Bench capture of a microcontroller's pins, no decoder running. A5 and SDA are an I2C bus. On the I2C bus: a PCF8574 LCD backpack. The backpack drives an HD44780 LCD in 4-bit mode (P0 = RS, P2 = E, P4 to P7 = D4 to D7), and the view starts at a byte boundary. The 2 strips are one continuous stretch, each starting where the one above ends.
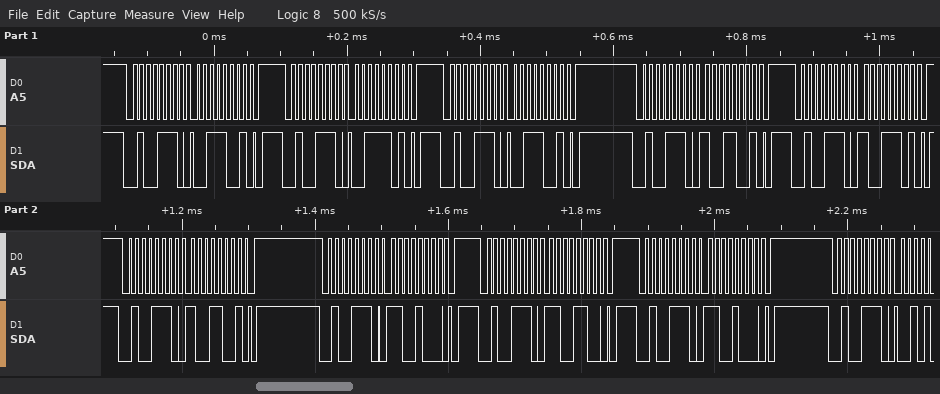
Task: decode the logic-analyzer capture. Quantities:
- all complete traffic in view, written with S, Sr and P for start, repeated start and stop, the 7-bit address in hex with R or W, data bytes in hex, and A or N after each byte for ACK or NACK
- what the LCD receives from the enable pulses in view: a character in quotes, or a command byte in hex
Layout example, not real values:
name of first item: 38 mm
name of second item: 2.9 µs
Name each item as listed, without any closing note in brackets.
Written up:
all complete traffic in view, written with S, Sr and P for start, repeated start and stop, the 7-bit address in hex with R or W, data bytes in hex, and A or N after each byte for ACK or NACK: S 27W A 39 A P S 27W A 3D A P S 27W A 39 A P S 27W A 99 A P S 27W A 9D A P S 27W A 99 A P S 27W A C8 A P S 27W A CC A P S 27W A C8 A P S 27W A
what the LCD receives from the enable pulses in view: a character in quotes, or a command byte in hex: '9'
